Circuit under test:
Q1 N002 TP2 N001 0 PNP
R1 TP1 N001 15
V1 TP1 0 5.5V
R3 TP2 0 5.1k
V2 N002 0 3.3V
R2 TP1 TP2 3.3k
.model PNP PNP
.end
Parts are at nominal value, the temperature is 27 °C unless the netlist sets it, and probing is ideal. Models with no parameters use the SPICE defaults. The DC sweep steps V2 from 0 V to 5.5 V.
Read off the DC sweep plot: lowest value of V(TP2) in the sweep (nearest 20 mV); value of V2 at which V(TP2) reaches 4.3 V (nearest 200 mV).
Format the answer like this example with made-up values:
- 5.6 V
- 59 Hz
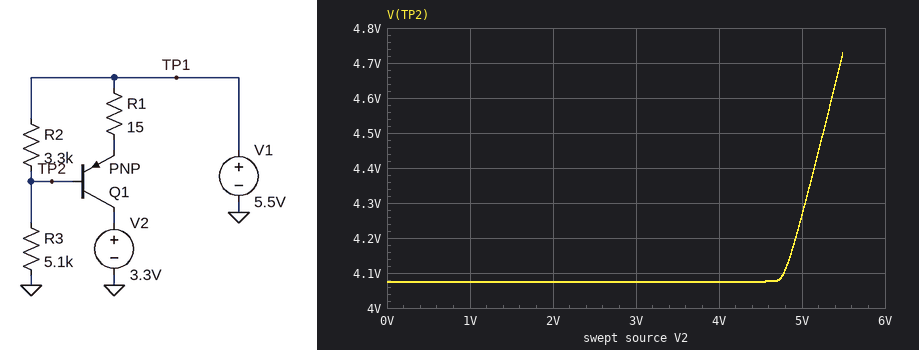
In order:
- 4.08 V
- 5.0 V
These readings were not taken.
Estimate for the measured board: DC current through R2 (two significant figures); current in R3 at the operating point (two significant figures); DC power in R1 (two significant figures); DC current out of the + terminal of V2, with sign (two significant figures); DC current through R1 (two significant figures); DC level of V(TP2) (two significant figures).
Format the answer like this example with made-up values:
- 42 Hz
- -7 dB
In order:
- 430 µA
- 800 µA
- 21 mW
- -37 mA
- 37 mA
- 4.1 V
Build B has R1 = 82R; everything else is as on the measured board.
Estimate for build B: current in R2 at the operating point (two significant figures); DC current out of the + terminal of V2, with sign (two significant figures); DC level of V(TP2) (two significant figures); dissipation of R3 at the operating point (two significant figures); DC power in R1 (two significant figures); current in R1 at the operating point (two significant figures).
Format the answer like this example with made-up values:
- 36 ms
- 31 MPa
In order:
- 580 µA
- -13 mA
- 3.6 V
- 2.5 mW
- 14 mW
- 13 mA
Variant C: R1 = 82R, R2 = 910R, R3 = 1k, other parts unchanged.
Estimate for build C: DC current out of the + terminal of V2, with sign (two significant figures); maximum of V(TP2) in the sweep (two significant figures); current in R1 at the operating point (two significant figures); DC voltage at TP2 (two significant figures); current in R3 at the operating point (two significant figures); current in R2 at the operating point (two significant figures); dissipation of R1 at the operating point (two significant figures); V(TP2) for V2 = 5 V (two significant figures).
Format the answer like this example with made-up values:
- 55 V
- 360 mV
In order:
- -20 mA
- 4.7 V
- 20 mA
- 3.0 V
- 3.0 mA
- 2.8 mA
- 34 mW
- 4.2 V
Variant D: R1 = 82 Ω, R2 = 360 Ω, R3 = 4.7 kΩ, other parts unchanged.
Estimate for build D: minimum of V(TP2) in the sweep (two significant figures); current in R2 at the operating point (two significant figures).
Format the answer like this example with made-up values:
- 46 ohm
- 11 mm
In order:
- 5.1 V
- 1.1 mA
